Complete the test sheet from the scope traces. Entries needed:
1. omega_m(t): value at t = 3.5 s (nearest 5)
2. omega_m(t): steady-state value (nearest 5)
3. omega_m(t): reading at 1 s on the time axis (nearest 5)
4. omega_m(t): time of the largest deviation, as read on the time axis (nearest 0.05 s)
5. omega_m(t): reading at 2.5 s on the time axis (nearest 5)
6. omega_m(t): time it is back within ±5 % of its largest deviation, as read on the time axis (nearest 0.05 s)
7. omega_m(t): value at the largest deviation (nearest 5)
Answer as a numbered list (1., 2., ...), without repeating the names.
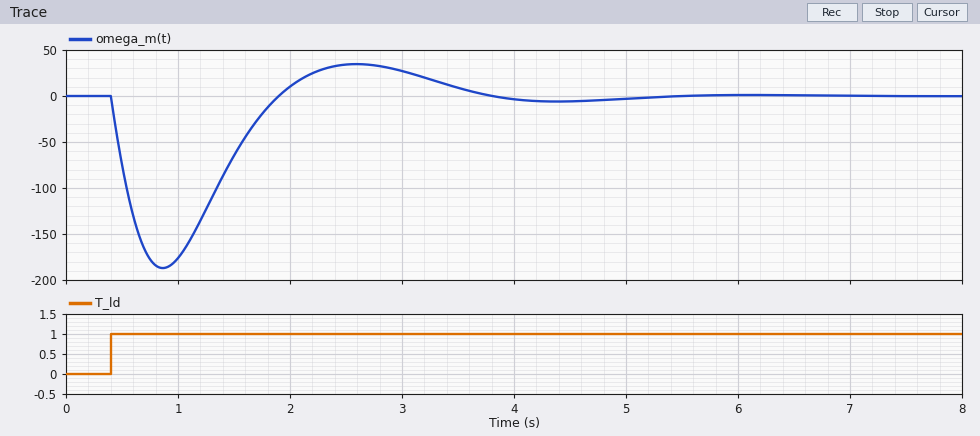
1. 10
2. 0
3. -175
4. 0.85 s
5. 35
6. 3.50 s
7. -185
